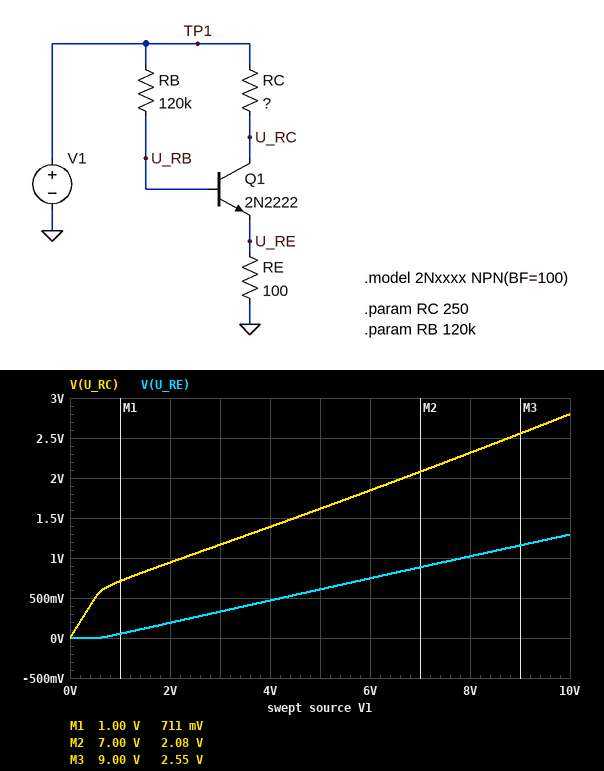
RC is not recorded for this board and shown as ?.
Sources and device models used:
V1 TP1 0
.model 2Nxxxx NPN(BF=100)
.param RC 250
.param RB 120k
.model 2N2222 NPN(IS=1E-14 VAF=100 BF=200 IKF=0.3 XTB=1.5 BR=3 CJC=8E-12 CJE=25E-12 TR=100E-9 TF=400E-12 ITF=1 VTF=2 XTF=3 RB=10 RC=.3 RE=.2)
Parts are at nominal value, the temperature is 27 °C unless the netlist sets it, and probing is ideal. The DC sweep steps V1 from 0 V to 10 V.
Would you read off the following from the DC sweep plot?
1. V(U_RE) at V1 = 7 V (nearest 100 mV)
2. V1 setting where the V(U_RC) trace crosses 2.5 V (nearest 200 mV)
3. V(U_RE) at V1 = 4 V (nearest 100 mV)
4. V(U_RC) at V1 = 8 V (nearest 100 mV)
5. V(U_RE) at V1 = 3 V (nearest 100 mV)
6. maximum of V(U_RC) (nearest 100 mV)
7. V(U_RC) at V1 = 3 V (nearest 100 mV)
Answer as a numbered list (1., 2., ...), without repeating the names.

1. 900 mV
2. 8.8 V
3. 500 mV
4. 2.3 V
5. 300 mV
6. 2.8 V
7. 1.2 V
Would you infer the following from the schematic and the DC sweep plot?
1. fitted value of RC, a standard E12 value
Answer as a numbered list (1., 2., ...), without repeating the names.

1. 560 Ω
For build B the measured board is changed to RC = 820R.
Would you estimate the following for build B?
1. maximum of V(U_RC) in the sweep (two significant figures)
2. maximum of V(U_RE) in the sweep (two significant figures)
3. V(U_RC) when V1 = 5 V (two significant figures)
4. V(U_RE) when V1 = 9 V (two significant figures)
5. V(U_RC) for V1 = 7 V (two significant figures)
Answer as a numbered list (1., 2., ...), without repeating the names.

1. 1.2 V
2. 1.1 V
3. 690 mV
4. 970 mV
5. 900 mV
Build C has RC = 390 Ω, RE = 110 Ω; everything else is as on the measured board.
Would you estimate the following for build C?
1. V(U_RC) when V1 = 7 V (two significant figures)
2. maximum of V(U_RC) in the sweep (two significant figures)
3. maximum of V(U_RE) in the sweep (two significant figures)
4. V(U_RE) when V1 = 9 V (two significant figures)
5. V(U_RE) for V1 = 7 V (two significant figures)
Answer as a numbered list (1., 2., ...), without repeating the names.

1. 3.6 V
2. 5.0 V
3. 1.4 V
4. 1.3 V
5. 970 mV
